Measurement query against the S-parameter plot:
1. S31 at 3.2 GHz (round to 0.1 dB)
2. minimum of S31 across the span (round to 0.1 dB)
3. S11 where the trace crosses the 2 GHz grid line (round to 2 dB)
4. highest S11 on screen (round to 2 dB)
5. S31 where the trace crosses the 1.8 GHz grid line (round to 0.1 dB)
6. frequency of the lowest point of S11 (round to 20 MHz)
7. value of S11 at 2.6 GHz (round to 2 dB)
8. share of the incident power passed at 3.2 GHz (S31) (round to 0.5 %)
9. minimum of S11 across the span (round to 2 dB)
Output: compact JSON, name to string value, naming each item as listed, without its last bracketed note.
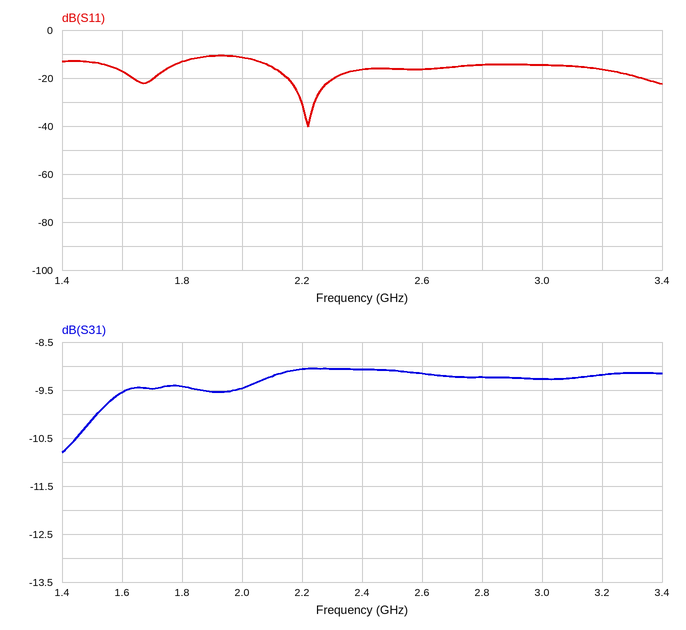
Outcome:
{"S31 at 3.2 GHz": "-9.2 dB", "minimum of S31 across the span": "-10.8 dB", "S11 where the trace crosses the 2 GHz grid line": "-12 dB", "highest S11 on screen": "-10 dB", "S31 where the trace crosses the 1.8 GHz grid line": "-9.4 dB", "frequency of the lowest point of S11": "2.22 GHz", "value of S11 at 2.6 GHz": "-16 dB", "share of the incident power passed at 3.2 GHz (S31)": "12.0 %", "minimum of S11 across the span": "-40 dB"}
